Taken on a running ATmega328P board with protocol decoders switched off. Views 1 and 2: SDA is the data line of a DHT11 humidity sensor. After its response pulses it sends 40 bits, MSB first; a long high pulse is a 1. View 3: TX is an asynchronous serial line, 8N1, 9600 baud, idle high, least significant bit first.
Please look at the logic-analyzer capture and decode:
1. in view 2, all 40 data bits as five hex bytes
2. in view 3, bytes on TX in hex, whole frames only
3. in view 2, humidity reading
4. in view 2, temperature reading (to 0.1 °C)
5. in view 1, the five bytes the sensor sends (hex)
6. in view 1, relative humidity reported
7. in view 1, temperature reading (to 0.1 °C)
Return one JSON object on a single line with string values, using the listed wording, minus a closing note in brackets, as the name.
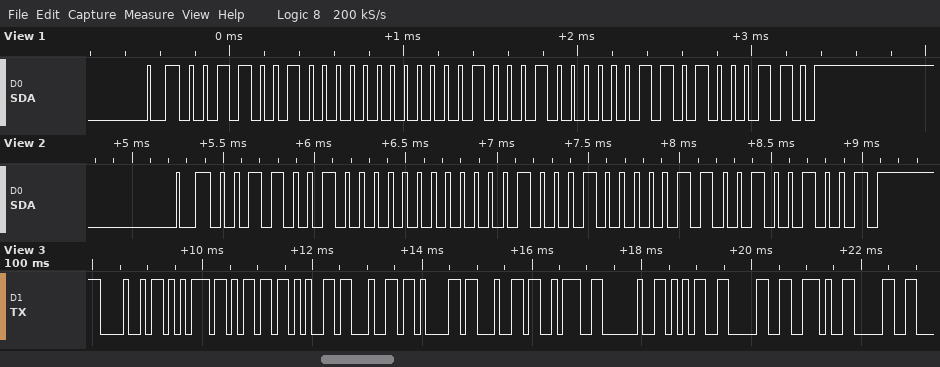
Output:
{"in view 2, all 40 data bits as five hex bytes": "32 00 11 06 49", "in view 3, bytes on TX in hex, whole frames only": "48 75 6D 65 64 61 64 3A 20 35 30 2E 30", "in view 2, humidity reading": "50 %", "in view 2, temperature reading": "17.6 °C", "in view 1, the five bytes the sensor sends": "32 00 11 03 46", "in view 1, relative humidity reported": "50 %", "in view 1, temperature reading": "17.3 °C"}
